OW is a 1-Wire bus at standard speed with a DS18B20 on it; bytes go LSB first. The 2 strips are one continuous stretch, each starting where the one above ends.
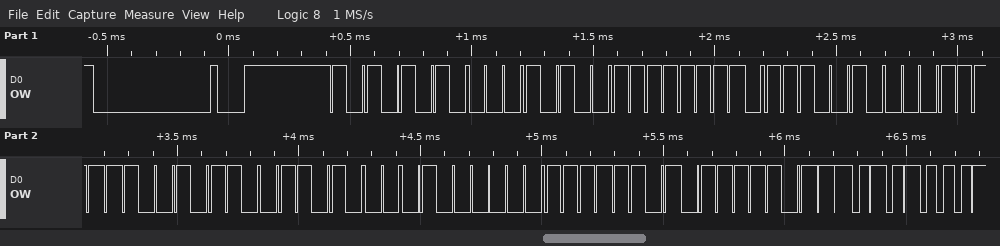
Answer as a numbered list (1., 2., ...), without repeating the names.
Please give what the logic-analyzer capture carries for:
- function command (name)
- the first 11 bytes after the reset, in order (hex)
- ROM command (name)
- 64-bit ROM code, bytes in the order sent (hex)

1. Read Scratchpad
2. 55 28 FF 4E F8 69 16 02 BF BE 2B
3. Match ROM
4. 28 FF 4E F8 69 16 02 BF
